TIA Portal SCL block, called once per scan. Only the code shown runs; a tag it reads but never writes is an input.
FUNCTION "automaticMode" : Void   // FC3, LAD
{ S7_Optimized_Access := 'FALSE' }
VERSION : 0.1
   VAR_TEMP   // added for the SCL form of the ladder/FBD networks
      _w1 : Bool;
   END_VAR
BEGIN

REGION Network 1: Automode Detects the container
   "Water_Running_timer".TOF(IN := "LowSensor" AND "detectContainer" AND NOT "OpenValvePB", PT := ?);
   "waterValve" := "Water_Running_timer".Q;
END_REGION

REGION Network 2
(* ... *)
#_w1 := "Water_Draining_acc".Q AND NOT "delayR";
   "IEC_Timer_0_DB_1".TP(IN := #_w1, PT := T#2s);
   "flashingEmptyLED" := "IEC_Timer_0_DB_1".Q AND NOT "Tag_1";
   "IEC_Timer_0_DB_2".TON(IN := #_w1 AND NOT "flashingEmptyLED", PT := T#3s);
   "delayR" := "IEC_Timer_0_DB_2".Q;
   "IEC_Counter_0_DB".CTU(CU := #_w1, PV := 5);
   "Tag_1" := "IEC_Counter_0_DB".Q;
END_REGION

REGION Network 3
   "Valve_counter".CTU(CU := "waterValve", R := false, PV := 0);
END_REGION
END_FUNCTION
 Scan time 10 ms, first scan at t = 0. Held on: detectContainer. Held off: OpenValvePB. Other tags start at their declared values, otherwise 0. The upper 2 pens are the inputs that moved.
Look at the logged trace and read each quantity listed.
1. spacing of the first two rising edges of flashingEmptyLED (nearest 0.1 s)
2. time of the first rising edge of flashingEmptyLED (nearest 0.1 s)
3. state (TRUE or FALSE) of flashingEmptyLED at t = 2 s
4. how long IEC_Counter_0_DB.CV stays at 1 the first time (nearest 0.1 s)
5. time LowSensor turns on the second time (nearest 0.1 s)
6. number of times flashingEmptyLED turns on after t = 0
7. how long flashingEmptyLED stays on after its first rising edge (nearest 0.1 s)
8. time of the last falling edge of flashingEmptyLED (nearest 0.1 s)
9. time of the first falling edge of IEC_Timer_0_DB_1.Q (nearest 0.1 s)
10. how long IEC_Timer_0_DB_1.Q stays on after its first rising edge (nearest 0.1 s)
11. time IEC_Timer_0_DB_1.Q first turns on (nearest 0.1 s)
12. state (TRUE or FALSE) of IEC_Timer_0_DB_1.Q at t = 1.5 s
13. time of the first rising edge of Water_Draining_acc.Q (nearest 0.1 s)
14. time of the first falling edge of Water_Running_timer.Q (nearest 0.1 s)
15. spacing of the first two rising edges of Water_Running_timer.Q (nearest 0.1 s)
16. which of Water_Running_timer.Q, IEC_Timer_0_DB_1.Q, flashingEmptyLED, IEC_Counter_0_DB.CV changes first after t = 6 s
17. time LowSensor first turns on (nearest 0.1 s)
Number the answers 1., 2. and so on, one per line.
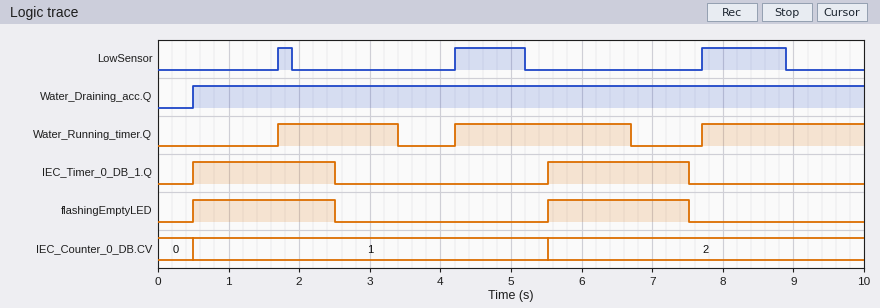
1. 5.0 s
2. 0.5 s
3. TRUE
4. 5.0 s
5. 4.2 s
6. 2
7. 2.0 s
8. 7.5 s
9. 2.5 s
10. 2.0 s
11. 0.5 s
12. TRUE
13. 0.5 s
14. 3.4 s
15. 2.5 s
16. Water_Running_timer.Q
17. 1.7 s
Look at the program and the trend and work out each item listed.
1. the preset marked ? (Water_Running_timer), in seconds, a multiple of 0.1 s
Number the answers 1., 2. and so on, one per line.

1. 1.5 s
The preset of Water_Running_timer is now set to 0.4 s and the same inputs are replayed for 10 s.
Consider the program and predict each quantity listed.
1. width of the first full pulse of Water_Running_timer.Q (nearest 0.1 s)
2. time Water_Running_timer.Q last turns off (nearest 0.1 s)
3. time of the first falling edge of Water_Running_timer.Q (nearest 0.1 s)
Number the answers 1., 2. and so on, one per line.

1. 0.6 s
2. 9.3 s
3. 2.3 s
